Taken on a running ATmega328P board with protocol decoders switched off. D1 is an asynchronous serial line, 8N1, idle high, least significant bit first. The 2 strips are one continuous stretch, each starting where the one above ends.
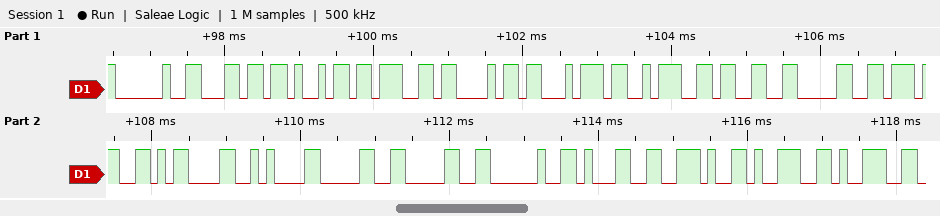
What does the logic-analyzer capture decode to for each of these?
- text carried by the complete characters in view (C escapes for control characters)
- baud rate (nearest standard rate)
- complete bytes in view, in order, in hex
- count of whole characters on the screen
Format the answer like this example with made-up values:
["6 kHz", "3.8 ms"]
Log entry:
["\" light:307\\r\\n00 1.99\"", "9600 baud", "20 6C 69 67 68 74 3A 33 30 37 0D 0A 30 30 20 31 2E 39 39", "19"]
